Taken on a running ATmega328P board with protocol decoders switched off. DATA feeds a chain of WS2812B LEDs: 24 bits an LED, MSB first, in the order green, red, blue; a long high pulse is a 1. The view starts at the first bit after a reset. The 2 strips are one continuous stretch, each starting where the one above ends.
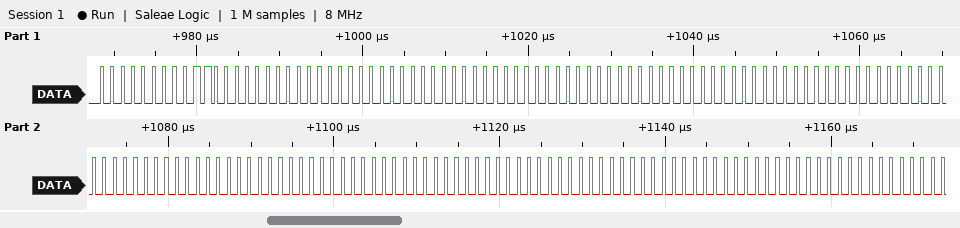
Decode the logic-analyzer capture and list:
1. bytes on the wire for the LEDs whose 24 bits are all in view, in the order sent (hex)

00 60 00 00 00 00 00 00 00 00 00 00 00 00 00 00 00 00
